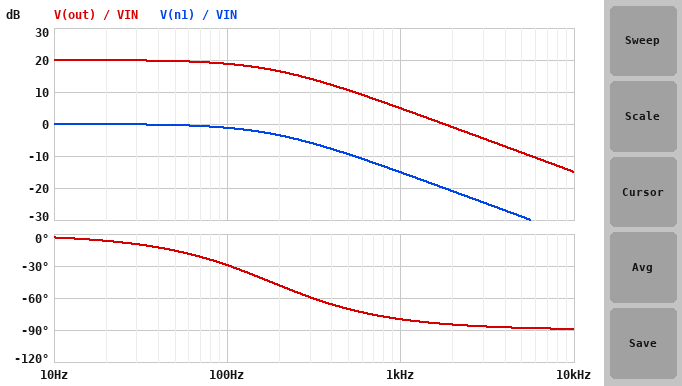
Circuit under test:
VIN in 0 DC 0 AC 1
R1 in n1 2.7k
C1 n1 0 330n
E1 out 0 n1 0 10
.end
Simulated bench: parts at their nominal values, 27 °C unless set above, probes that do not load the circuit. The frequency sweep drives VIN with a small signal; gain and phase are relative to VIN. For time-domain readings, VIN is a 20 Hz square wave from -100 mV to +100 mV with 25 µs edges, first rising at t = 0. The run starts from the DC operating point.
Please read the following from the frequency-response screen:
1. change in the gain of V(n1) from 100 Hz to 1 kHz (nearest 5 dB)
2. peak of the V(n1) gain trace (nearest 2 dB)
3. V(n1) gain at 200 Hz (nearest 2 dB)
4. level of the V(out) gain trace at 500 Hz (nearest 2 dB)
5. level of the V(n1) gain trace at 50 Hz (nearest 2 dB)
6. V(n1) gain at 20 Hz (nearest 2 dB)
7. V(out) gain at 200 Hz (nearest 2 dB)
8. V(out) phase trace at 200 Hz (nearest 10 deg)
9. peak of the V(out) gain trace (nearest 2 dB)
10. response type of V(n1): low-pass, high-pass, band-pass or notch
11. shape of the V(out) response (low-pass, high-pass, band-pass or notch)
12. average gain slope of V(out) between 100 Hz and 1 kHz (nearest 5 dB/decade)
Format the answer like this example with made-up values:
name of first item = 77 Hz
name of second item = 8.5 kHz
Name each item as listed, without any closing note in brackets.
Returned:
change in the gain of V(n1) from 100 Hz to 1 kHz = -15 dB
peak of the V(n1) gain trace = 0 dB
V(n1) gain at 200 Hz = -4 dB
level of the V(out) gain trace at 500 Hz = 10 dB
level of the V(n1) gain trace at 50 Hz = 0 dB
V(n1) gain at 20 Hz = 0 dB
V(out) gain at 200 Hz = 16 dB
V(out) phase trace at 200 Hz = -50 deg
peak of the V(out) gain trace = 20 dB
response type of V(n1): low-pass, high-pass, band-pass or notch = low-pass
shape of the V(out) response = low-pass
average gain slope of V(out) between 100 Hz and 1 kHz = -15 dB/decade
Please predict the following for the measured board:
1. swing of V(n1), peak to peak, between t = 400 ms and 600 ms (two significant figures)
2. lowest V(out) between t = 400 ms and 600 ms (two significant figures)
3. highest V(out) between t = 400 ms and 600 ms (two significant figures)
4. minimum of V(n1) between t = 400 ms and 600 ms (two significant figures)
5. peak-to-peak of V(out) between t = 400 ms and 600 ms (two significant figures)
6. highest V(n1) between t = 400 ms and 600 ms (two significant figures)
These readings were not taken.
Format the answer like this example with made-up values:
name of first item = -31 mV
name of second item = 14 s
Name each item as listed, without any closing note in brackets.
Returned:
swing of V(n1), peak to peak, between t = 400 ms and 600 ms = 200 mV
lowest V(out) between t = 400 ms and 600 ms = -1.0 V
highest V(out) between t = 400 ms and 600 ms = 1.0 V
minimum of V(n1) between t = 400 ms and 600 ms = -100 mV
peak-to-peak of V(out) between t = 400 ms and 600 ms = 2.0 V
highest V(n1) between t = 400 ms and 600 ms = 100 mV
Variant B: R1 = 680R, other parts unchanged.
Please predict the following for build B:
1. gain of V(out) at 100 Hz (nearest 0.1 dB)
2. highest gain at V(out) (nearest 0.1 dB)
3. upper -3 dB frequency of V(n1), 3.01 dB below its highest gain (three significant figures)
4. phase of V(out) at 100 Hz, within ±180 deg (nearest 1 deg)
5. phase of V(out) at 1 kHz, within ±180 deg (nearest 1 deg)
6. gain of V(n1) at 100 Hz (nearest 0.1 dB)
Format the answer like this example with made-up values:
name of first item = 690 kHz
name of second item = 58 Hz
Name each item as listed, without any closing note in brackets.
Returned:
gain of V(out) at 100 Hz = 19.9 dB
highest gain at V(out) = 20.0 dB
upper -3 dB frequency of V(n1), 3.01 dB below its highest gain = 709 Hz
phase of V(out) at 100 Hz, within ±180 deg = -8 deg
phase of V(out) at 1 kHz, within ±180 deg = -55 deg
gain of V(n1) at 100 Hz = -0.1 dB
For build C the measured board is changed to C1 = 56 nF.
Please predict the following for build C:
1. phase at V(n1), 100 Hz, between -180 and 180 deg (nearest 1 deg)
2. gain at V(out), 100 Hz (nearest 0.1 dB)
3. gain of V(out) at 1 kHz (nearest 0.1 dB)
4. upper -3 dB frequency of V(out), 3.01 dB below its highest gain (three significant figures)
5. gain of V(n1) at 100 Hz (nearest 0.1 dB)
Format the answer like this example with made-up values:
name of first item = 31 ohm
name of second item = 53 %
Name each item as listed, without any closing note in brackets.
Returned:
phase at V(n1), 100 Hz, between -180 and 180 deg = -5 deg
gain at V(out), 100 Hz = 20.0 dB
gain of V(out) at 1 kHz = 17.2 dB
upper -3 dB frequency of V(out), 3.01 dB below its highest gain = 1.05 kHz
gain of V(n1) at 100 Hz = 0 dB
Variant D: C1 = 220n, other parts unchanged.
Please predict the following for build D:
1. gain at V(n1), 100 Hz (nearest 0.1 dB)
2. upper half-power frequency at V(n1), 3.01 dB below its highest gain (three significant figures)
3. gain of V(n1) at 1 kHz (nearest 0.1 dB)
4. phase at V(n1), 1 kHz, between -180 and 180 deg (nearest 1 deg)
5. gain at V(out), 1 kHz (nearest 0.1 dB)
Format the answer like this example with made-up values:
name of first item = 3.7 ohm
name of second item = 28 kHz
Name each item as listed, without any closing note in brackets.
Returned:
gain at V(n1), 100 Hz = -0.6 dB
upper half-power frequency at V(n1), 3.01 dB below its highest gain = 268 Hz
gain of V(n1) at 1 kHz = -11.7 dB
phase at V(n1), 1 kHz, between -180 and 180 deg = -75 deg
gain at V(out), 1 kHz = 8.3 dB
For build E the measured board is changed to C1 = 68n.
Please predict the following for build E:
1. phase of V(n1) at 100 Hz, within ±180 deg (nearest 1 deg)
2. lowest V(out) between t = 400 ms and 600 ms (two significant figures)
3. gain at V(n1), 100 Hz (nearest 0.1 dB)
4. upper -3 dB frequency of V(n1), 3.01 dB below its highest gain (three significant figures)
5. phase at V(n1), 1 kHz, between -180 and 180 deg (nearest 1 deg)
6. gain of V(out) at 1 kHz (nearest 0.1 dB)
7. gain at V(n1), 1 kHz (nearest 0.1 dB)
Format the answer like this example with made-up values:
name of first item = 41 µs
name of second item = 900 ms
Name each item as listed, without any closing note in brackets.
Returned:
phase of V(n1) at 100 Hz, within ±180 deg = -7 deg
lowest V(out) between t = 400 ms and 600 ms = -1.0 V
gain at V(n1), 100 Hz = -0.1 dB
upper -3 dB frequency of V(n1), 3.01 dB below its highest gain = 867 Hz
phase at V(n1), 1 kHz, between -180 and 180 deg = -49 deg
gain of V(out) at 1 kHz = 16.3 dB
gain at V(n1), 1 kHz = -3.7 dB
